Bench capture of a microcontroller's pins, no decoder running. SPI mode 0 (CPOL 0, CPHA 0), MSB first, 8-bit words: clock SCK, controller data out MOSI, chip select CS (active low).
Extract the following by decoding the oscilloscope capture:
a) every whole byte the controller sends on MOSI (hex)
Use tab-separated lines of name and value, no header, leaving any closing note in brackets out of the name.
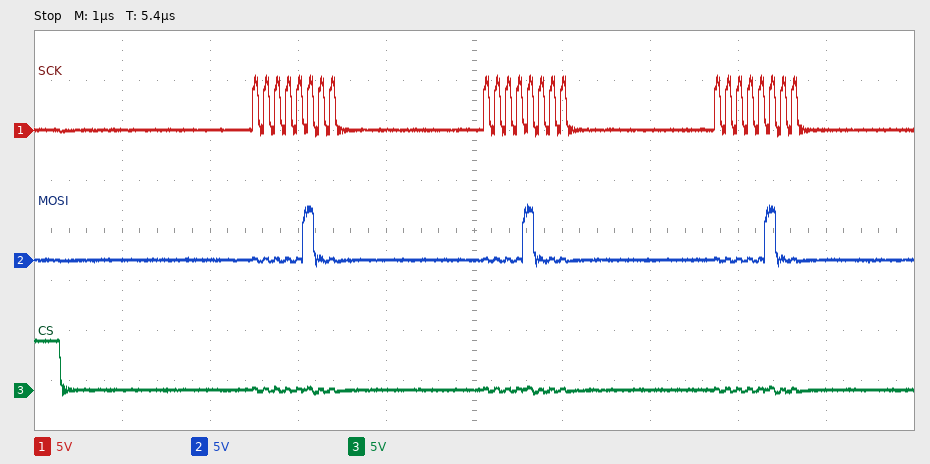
every whole byte the controller sends on MOSI	0x04 0x08 0x04
